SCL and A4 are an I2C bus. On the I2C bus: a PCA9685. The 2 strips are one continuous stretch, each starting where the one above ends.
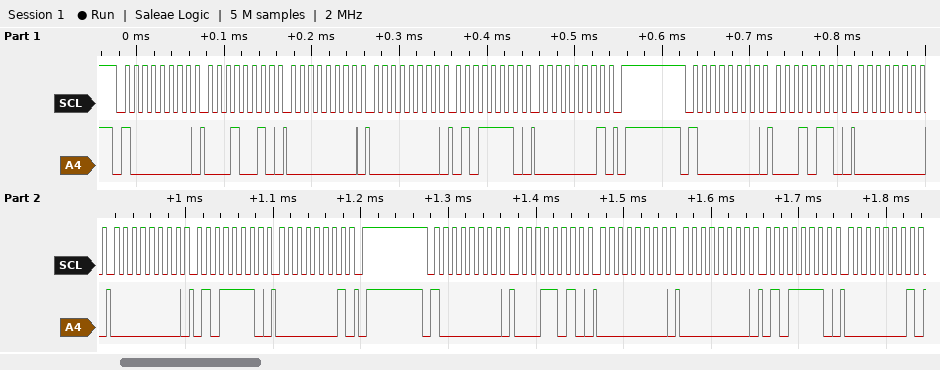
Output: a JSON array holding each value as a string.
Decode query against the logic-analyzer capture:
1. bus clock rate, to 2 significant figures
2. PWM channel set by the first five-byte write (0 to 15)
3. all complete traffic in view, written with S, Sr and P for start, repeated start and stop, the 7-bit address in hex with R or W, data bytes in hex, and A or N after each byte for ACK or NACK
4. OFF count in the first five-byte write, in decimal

["100 kHz", "3", "S 40W A 12 A 00 A 00 A 5E A 01 A P S 40W A 16 A 00 A 00 A 5E A 01 A P S 40W A 1A A 00 A 00 A 5E A 01 A", "350"]
